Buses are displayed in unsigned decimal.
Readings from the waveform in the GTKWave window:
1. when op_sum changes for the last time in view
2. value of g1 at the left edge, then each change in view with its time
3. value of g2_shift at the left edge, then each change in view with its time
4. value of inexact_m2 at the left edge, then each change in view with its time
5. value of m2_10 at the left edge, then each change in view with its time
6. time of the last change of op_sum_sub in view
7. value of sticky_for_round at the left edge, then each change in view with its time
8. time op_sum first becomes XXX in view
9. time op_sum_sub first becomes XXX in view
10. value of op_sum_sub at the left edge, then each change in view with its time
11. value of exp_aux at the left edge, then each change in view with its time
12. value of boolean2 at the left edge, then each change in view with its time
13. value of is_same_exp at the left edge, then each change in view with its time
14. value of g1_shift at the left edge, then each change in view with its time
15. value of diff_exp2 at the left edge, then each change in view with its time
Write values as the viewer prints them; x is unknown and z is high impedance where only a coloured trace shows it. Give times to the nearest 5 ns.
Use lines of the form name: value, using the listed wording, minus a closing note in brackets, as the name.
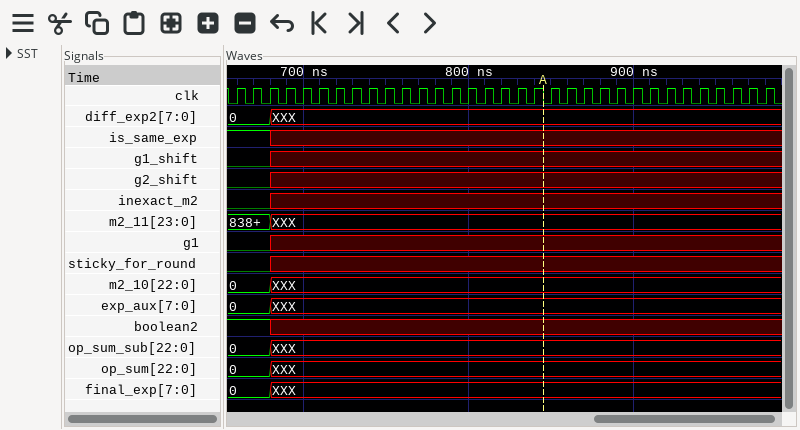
when op_sum changes for the last time in view: 680 ns
value of g1 at the left edge, then each change in view with its time: 0, x at 680 ns
value of g2_shift at the left edge, then each change in view with its time: 0, x at 680 ns
value of inexact_m2 at the left edge, then each change in view with its time: 0, x at 680 ns
value of m2_10 at the left edge, then each change in view with its time: 0, XXX at 680 ns
time of the last change of op_sum_sub in view: 680 ns
value of sticky_for_round at the left edge, then each change in view with its time: 0, x at 680 ns
time op_sum first becomes XXX in view: 680 ns
time op_sum_sub first becomes XXX in view: 680 ns
value of op_sum_sub at the left edge, then each change in view with its time: 0, XXX at 680 ns
value of exp_aux at the left edge, then each change in view with its time: 0, XXX at 680 ns
value of boolean2 at the left edge, then each change in view with its time: 1, x at 680 ns
value of is_same_exp at the left edge, then each change in view with its time: 1, x at 680 ns
value of g1_shift at the left edge, then each change in view with its time: 0, x at 680 ns
value of diff_exp2 at the left edge, then each change in view with its time: 0, XXX at 680 ns
